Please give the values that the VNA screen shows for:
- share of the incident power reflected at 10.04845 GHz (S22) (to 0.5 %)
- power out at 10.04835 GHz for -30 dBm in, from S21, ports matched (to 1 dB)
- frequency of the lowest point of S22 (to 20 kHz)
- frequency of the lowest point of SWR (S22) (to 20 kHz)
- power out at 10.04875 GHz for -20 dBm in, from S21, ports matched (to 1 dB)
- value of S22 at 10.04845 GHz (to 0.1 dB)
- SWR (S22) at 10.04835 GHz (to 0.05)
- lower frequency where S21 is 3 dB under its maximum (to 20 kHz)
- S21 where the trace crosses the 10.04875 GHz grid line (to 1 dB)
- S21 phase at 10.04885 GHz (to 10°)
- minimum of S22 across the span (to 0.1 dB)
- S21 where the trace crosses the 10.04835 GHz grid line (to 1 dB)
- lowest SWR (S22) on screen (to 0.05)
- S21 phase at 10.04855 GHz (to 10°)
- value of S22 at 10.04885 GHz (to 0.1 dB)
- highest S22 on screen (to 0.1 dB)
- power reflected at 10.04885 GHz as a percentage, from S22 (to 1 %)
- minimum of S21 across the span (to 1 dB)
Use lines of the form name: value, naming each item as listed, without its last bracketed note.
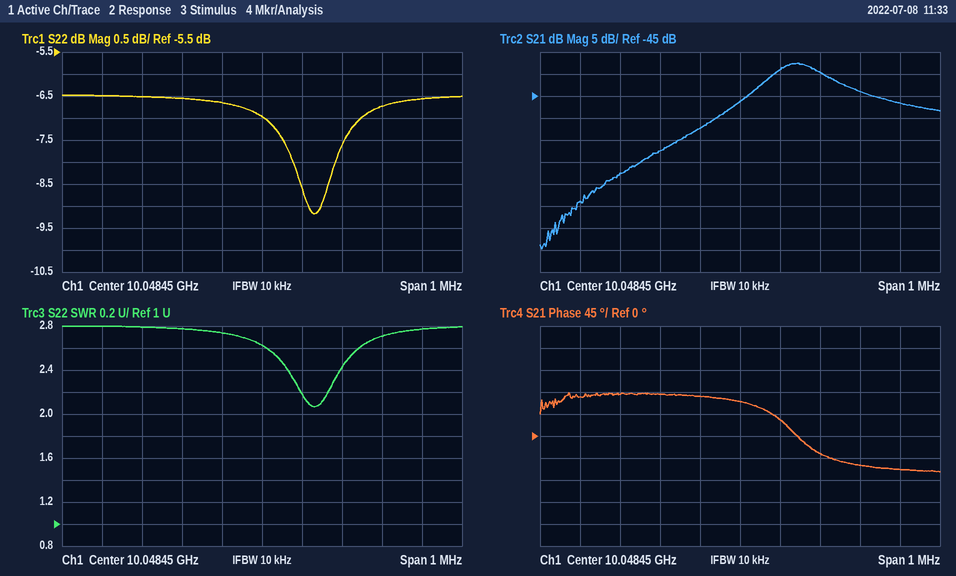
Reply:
share of the incident power reflected at 10.04845 GHz (S22): 20.0 %
power out at 10.04835 GHz for -30 dBm in, from S21, ports matched: -82 dBm
frequency of the lowest point of S22: 10.04858 GHz
frequency of the lowest point of SWR (S22): 10.04858 GHz
power out at 10.04875 GHz for -20 dBm in, from S21, ports matched: -64 dBm
value of S22 at 10.04845 GHz: -7.0 dB
SWR (S22) at 10.04835 GHz: 2.75
lower frequency where S21 is 3 dB under its maximum: 10.04852 GHz
S21 where the trace crosses the 10.04875 GHz grid line: -44 dB
S21 phase at 10.04885 GHz: -70°
minimum of S22 across the span: -9.2 dB
S21 where the trace crosses the 10.04835 GHz grid line: -52 dB
lowest SWR (S22) on screen: 2.05
S21 phase at 10.04855 GHz: 30°
value of S22 at 10.04885 GHz: -6.6 dB
highest S22 on screen: -6.5 dB
power reflected at 10.04885 GHz as a percentage, from S22: 22 %
minimum of S21 across the span: -80 dB
